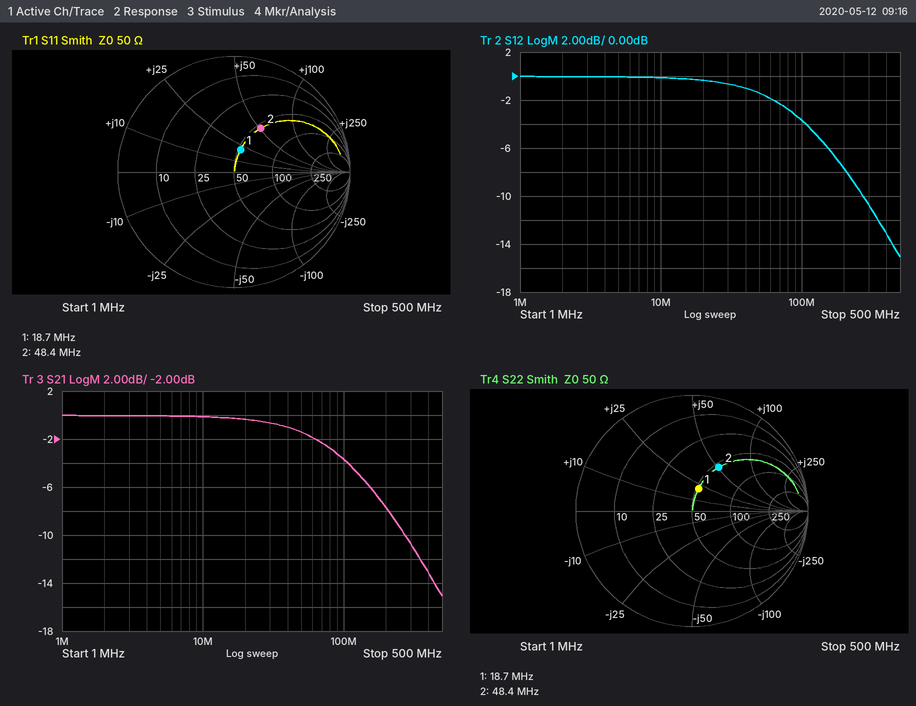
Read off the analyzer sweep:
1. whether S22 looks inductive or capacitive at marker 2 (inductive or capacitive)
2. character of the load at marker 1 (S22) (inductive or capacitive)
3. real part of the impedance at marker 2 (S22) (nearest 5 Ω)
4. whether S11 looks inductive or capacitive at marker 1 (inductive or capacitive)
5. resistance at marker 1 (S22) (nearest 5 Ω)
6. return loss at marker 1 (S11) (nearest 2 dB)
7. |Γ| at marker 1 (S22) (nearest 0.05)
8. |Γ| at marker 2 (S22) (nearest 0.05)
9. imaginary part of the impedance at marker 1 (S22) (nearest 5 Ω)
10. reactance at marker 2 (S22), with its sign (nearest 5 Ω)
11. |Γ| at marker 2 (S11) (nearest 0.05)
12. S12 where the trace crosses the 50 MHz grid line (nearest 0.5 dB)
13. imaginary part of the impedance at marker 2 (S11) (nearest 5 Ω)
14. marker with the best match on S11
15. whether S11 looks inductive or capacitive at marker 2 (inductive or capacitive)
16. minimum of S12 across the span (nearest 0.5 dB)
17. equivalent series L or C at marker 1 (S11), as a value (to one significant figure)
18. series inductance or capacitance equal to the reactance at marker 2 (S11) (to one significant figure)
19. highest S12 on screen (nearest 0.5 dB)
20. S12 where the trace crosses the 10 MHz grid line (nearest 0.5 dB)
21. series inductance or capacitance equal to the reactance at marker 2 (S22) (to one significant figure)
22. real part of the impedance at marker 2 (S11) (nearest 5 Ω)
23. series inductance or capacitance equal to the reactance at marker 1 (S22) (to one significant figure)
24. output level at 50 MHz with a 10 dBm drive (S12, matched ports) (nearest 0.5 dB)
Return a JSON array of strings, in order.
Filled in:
["inductive", "inductive", "55 Ω", "inductive", "50 Ω", "14 dB", "0.20", "0.45", "+20 Ω", "+50 Ω", "0.45", "-1.5 dB", "+50 Ω", "marker 1", "inductive", "-15.0 dB", "200 nH", "200 nH", "0.0 dB", "0.0 dB", "200 nH", "55 Ω", "200 nH", "8.5 dBm"]
